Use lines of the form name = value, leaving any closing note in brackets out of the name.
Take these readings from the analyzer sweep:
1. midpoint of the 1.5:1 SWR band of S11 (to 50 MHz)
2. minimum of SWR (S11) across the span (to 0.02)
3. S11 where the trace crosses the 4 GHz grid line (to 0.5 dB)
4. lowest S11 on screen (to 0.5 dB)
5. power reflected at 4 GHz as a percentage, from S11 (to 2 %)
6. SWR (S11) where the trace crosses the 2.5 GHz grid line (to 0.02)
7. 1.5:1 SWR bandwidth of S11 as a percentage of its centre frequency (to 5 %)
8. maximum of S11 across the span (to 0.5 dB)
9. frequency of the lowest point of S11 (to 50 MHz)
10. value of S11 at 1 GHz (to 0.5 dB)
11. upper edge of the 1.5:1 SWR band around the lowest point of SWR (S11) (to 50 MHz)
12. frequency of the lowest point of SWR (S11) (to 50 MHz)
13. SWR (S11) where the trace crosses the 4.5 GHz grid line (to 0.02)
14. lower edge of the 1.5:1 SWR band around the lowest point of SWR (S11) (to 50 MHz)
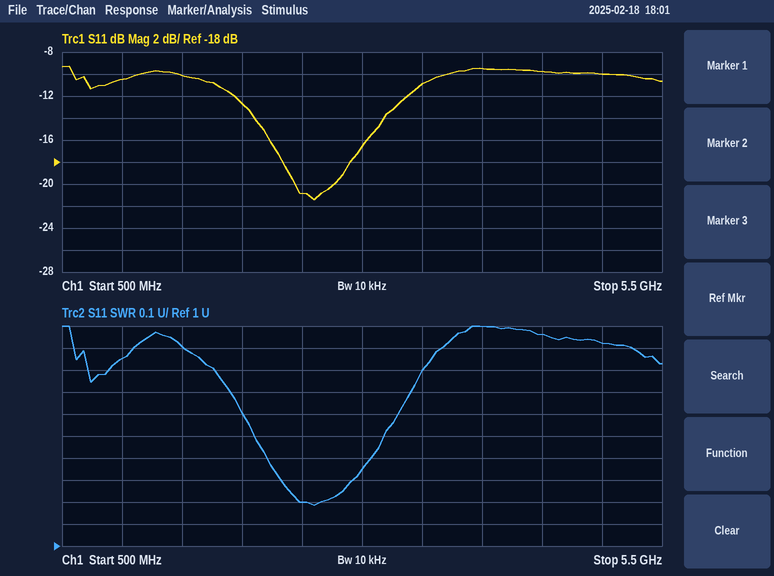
midpoint of the 1.5:1 SWR band of S11 = 2.65 GHz
minimum of SWR (S11) across the span = 1.18
S11 where the trace crosses the 4 GHz grid line = -9.5 dB
lowest S11 on screen = -21.5 dB
power reflected at 4 GHz as a percentage, from S11 = 12 %
SWR (S11) where the trace crosses the 2.5 GHz grid line = 1.20
1.5:1 SWR bandwidth of S11 as a percentage of its centre frequency = 40 %
maximum of S11 across the span = -9.5 dB
frequency of the lowest point of S11 = 2.60 GHz
value of S11 at 1 GHz = -10.5 dB
upper edge of the 1.5:1 SWR band around the lowest point of SWR (S11) = 3.20 GHz
frequency of the lowest point of SWR (S11) = 2.60 GHz
SWR (S11) where the trace crosses the 4.5 GHz grid line = 1.96
lower edge of the 1.5:1 SWR band around the lowest point of SWR (S11) = 2.10 GHz
